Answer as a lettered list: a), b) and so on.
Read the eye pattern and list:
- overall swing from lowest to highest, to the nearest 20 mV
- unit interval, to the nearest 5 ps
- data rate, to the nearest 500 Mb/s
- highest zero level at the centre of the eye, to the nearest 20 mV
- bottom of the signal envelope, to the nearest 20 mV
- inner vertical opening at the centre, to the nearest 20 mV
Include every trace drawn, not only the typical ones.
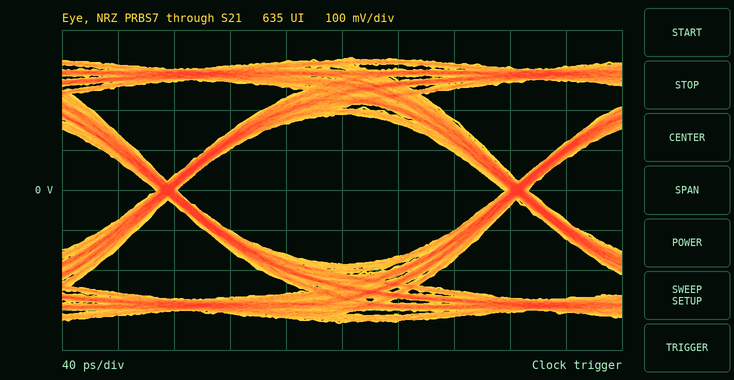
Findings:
a) 660 mV
b) 250 ps
c) 4.0 Gb/s
d) -180 mV
e) -340 mV
f) 380 mV
